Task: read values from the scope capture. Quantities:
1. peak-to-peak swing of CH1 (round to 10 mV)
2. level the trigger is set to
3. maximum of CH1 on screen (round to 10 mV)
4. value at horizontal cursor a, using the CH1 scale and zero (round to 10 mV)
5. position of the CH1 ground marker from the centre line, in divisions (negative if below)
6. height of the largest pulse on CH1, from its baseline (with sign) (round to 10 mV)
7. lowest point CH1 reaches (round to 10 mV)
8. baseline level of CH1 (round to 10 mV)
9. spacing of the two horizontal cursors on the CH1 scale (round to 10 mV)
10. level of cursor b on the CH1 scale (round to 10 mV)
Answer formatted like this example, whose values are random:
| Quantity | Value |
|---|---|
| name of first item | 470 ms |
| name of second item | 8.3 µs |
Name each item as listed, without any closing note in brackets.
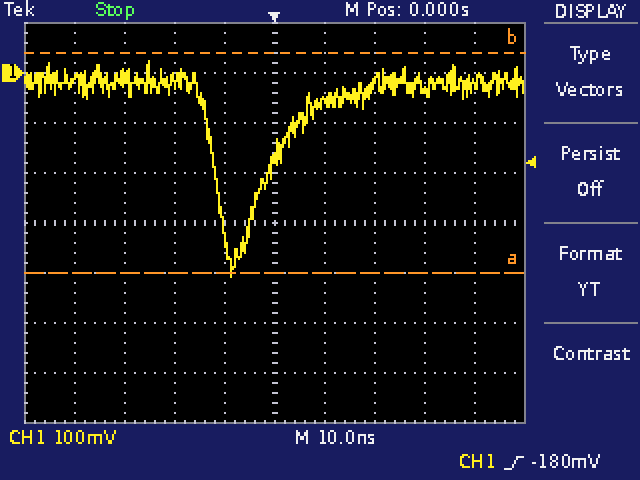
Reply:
| Quantity | Value |
|---|---|
| peak-to-peak swing of CH1 | 430 mV |
| level the trigger is set to | -180 mV |
| maximum of CH1 on screen | 20 mV |
| value at horizontal cursor a, using the CH1 scale and zero | -400 mV |
| position of the CH1 ground marker from the centre line, in divisions | +3.0 div |
| height of the largest pulse on CH1, from its baseline (with sign) | -390 mV |
| lowest point CH1 reaches | -410 mV |
| baseline level of CH1 | -20 mV |
| spacing of the two horizontal cursors on the CH1 scale | 440 mV |
| level of cursor b on the CH1 scale | 40 mV |
